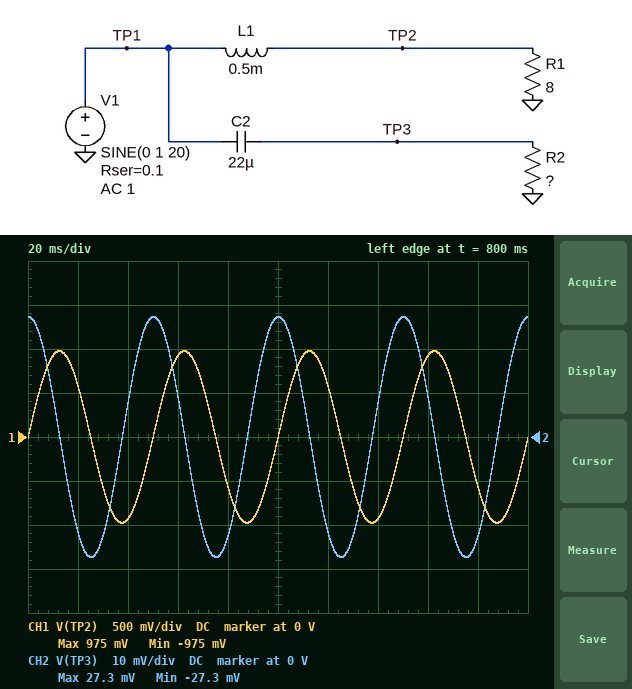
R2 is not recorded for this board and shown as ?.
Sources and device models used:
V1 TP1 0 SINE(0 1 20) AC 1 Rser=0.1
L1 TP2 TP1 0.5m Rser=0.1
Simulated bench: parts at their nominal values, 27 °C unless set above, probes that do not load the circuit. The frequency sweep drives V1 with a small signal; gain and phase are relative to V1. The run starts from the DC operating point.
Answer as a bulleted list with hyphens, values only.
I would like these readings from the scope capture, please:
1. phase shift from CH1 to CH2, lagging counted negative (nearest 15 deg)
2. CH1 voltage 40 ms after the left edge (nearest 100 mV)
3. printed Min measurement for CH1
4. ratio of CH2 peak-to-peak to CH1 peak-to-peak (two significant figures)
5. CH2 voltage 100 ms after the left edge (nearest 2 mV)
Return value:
- 90 deg
- -900 mV
- -975 mV
- 0.028
- 28 mV
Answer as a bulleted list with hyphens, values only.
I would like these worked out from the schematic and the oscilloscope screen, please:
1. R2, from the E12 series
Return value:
- 10 Ω
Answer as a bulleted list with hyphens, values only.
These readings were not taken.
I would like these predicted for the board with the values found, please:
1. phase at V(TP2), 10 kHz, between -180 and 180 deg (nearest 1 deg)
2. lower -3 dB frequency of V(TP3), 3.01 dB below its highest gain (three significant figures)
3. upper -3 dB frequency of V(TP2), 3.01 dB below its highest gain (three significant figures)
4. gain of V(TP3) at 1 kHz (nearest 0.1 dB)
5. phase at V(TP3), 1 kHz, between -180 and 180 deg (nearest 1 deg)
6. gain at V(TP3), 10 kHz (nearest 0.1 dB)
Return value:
- -75 deg
- 733 Hz
- 2.56 kHz
- -2.0 dB
- 36 deg
- -0.1 dB
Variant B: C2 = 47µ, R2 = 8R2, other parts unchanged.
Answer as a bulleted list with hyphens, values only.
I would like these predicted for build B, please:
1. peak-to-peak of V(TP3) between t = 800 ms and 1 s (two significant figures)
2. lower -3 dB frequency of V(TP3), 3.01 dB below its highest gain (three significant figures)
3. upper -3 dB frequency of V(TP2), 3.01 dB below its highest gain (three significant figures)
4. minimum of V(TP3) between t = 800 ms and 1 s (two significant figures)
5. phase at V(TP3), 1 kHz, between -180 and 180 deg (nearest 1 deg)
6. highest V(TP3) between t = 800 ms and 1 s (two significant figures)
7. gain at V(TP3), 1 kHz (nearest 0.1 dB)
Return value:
- 96 mV
- 418 Hz
- 2.55 kHz
- -48 mV
- 22 deg
- 48 mV
- -0.9 dB
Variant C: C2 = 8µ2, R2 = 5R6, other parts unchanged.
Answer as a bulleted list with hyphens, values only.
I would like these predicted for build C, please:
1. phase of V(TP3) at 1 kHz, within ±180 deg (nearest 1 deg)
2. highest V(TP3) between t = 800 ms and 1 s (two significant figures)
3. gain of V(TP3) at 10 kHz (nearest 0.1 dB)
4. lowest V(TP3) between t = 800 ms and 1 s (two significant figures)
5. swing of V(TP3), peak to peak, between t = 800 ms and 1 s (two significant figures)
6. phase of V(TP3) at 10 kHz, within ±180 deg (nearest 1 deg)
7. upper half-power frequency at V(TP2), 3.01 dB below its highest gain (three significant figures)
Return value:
- 74 deg
- 5.7 mV
- -0.6 dB
- -5.7 mV
- 11 mV
- 19 deg
- 2.58 kHz
